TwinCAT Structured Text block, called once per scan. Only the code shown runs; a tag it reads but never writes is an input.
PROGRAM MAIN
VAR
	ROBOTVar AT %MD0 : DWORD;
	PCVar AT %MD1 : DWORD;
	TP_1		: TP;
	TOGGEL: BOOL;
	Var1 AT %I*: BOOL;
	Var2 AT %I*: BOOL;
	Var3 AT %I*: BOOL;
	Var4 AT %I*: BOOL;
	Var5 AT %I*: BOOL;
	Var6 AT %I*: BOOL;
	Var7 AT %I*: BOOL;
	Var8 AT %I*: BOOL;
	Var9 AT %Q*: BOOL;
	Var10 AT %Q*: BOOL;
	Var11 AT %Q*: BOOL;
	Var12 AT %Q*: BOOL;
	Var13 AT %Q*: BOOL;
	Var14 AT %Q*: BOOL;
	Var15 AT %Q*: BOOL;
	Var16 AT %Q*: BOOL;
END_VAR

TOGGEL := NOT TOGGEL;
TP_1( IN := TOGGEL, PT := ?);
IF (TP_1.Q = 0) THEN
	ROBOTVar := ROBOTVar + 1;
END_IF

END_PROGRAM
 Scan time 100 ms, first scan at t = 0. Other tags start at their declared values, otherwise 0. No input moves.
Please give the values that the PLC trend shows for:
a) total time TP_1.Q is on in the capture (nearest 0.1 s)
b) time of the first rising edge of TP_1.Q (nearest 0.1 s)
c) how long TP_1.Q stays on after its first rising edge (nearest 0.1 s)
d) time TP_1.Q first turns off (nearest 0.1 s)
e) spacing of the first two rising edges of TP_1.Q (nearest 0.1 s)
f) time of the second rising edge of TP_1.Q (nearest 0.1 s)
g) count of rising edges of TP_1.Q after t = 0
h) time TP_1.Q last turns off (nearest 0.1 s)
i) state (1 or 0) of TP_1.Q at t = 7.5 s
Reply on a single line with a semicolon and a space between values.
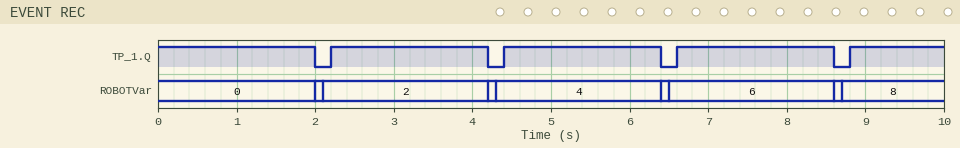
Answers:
9.2 s; 2.2 s; 2.0 s; 2.0 s; 2.2 s; 4.4 s; 4; 8.6 s; 1
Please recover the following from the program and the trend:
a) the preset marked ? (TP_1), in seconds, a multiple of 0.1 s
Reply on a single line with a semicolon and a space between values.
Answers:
2.0 s
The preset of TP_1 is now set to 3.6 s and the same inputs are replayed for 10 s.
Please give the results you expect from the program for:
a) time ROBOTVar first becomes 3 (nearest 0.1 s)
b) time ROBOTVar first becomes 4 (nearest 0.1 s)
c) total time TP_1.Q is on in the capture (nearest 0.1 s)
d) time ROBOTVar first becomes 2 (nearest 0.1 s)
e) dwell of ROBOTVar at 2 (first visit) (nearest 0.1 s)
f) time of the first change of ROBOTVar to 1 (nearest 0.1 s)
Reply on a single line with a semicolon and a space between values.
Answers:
7.4 s; 7.5 s; 9.6 s; 3.7 s; 3.7 s; 3.6 s
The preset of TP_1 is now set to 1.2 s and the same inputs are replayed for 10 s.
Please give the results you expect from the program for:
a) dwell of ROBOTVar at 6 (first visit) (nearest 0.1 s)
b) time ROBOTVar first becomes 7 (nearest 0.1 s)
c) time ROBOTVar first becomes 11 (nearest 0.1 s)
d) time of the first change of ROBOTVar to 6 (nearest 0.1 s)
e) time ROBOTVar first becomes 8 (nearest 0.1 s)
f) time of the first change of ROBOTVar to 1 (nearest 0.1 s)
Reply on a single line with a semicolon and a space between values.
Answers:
1.3 s; 5.4 s; 8.2 s; 4.1 s; 5.5 s; 1.2 s
